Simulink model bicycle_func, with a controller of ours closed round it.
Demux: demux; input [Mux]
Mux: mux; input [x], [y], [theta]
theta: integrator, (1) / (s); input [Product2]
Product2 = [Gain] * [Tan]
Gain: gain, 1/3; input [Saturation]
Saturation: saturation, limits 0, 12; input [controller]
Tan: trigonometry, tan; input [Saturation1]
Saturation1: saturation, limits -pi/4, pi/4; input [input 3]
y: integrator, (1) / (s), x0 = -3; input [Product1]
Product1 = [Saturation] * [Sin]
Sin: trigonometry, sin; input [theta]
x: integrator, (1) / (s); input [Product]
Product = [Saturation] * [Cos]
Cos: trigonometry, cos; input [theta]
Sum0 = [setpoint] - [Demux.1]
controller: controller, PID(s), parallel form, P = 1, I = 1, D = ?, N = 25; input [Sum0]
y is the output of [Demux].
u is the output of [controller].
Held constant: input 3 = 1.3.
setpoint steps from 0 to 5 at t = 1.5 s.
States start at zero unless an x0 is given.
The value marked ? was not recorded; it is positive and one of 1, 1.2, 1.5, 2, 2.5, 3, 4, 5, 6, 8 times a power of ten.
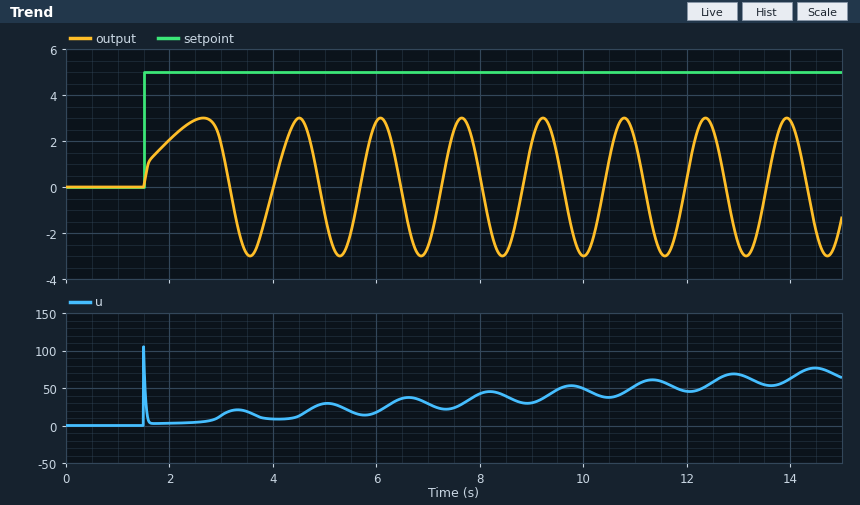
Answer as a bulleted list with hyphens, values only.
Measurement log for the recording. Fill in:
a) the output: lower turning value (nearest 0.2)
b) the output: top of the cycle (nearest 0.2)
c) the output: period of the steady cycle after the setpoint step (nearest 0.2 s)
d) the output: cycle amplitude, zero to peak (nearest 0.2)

- -3.0
- 3.0
- 1.6 s
- 3.0
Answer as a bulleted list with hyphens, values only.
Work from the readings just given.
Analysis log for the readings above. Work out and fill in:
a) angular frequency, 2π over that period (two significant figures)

- 3.9 rad/s
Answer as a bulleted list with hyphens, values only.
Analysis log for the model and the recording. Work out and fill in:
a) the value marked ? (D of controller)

- 0.8
